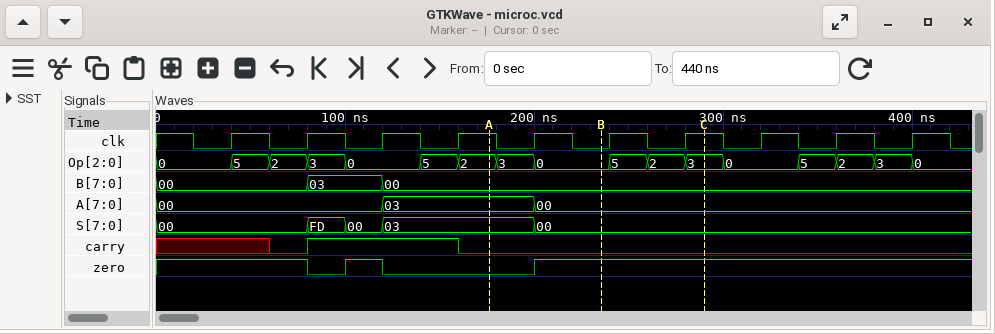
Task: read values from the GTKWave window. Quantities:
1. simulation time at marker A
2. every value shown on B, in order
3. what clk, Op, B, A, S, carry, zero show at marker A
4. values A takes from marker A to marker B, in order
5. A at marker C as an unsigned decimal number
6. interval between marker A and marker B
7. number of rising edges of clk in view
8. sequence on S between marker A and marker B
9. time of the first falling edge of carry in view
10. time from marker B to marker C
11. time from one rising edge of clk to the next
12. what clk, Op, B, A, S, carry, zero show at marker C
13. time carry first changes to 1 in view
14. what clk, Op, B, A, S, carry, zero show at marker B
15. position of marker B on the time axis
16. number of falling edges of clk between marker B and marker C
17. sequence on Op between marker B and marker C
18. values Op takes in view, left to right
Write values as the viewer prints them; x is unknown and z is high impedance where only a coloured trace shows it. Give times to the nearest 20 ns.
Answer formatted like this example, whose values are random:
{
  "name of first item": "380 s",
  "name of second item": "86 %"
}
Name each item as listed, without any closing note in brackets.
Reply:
{
  "simulation time at marker A": "180 ns",
  "every value shown on B, in order": "00, 03, 00",
  "what clk, Op, B, A, S, carry, zero show at marker A": "clk=1, Op=2, B=00, A=03, S=03, carry=0, zero=0",
  "values A takes from marker A to marker B, in order": "03, 00",
  "A at marker C as an unsigned decimal number": "0",
  "interval between marker A and marker B": "60 ns",
  "number of rising edges of clk in view": "10",
  "sequence on S between marker A and marker B": "03, 00",
  "time of the first falling edge of carry in view": "160 ns",
  "time from marker B to marker C": "60 ns",
  "time from one rising edge of clk to the next": "40 ns",
  "what clk, Op, B, A, S, carry, zero show at marker C": "clk=1, Op=3, B=00, A=00, S=00, carry=0, zero=1",
  "time carry first changes to 1 in view": "80 ns",
  "what clk, Op, B, A, S, carry, zero show at marker B": "clk=0, Op=0, B=00, A=00, S=00, carry=0, zero=1",
  "position of marker B on the time axis": "240 ns",
  "number of falling edges of clk between marker B and marker C": "1",
  "sequence on Op between marker B and marker C": "0, 5, 2, 3",
  "values Op takes in view, left to right": "0, 5, 2, 3, 0, 5, 2, 3, 0, 5, 2, 3, 0, 5, 2, 3, 0"
}
